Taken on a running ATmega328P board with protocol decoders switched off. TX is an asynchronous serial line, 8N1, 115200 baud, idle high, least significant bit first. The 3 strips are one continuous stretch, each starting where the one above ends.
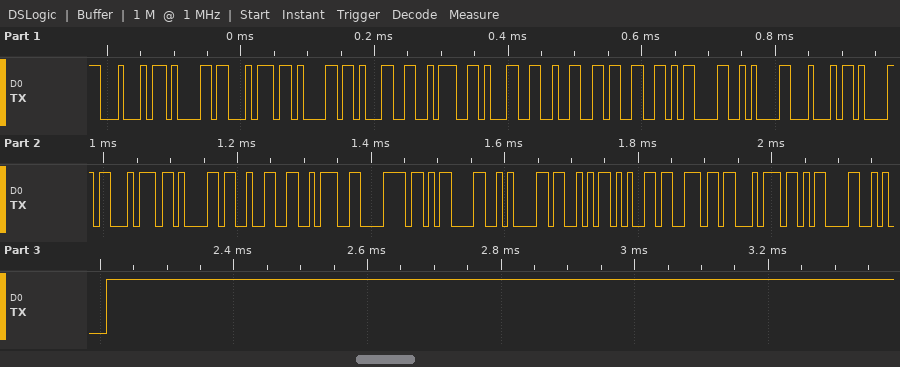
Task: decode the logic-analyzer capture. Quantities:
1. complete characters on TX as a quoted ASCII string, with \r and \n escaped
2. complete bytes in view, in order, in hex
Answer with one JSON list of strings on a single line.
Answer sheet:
["\"Data1:123\\r\\nData2:x\\r\\nSent\\r\\n\"", "0x44 0x61 0x74 0x61 0x31 0x3A 0x31 0x32 0x33 0x0D 0x0A 0x44 0x61 0x74 0x61 0x32 0x3A 0x78 0x0D 0x0A 0x53 0x65 0x6E 0x74 0x0D 0x0A"]
